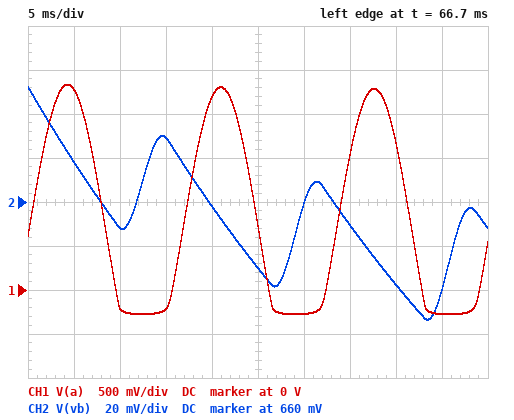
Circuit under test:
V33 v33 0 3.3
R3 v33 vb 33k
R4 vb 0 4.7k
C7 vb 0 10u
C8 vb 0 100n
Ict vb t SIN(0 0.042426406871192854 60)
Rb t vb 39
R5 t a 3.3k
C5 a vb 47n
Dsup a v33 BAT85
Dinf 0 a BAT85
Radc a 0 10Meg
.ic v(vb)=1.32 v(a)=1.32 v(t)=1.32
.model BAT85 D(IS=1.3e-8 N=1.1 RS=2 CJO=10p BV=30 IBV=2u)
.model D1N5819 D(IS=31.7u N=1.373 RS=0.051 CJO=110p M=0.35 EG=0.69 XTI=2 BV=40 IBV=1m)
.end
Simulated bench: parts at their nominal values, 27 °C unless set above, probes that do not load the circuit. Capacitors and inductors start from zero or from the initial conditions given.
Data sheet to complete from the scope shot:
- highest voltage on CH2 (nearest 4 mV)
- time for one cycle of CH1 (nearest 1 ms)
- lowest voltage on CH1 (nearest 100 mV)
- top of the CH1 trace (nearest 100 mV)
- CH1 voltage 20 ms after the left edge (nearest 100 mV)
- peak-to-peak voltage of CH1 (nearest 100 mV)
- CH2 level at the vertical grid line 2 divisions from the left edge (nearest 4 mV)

712 mV
17 ms
-300 mV
2.3 V
2.2 V
2.6 V
648 mV
